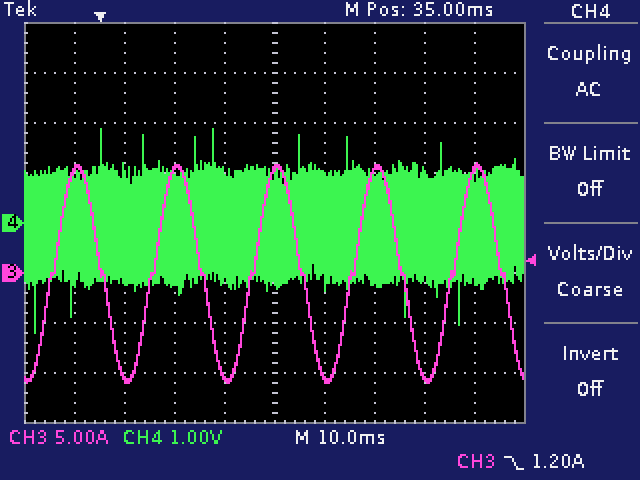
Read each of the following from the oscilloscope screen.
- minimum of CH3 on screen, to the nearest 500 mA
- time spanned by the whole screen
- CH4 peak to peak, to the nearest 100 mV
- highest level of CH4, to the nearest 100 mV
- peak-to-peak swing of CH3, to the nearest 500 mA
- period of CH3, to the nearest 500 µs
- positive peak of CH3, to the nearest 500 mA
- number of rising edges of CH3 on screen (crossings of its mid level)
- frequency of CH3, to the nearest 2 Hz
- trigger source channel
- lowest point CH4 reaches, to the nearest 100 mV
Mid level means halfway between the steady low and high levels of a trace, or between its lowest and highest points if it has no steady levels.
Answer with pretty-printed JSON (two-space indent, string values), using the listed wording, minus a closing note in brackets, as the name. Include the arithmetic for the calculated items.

{
  "minimum of CH3 on screen, to the nearest 500 mA": "-11.0 A",
  "time spanned by the whole screen": "100 ms",
  "CH4 peak to peak, to the nearest 100 mV": "1.9 V − (-2.2 V) = 4.1 V",
  "highest level of CH4, to the nearest 100 mV": "1.9 V",
  "peak-to-peak swing of CH3, to the nearest 500 mA": "11.0 A − (-11.0 A) = 22.0 A",
  "period of CH3, to the nearest 500 µs": "20.0 ms",
  "positive peak of CH3, to the nearest 500 mA": "11.0 A",
  "number of rising edges of CH3 on screen": "5",
  "frequency of CH3, to the nearest 2 Hz": "1 / 20.0 ms ≈ 50 Hz",
  "trigger source channel": "CH3",
  "lowest point CH4 reaches, to the nearest 100 mV": "-2.2 V"
}
